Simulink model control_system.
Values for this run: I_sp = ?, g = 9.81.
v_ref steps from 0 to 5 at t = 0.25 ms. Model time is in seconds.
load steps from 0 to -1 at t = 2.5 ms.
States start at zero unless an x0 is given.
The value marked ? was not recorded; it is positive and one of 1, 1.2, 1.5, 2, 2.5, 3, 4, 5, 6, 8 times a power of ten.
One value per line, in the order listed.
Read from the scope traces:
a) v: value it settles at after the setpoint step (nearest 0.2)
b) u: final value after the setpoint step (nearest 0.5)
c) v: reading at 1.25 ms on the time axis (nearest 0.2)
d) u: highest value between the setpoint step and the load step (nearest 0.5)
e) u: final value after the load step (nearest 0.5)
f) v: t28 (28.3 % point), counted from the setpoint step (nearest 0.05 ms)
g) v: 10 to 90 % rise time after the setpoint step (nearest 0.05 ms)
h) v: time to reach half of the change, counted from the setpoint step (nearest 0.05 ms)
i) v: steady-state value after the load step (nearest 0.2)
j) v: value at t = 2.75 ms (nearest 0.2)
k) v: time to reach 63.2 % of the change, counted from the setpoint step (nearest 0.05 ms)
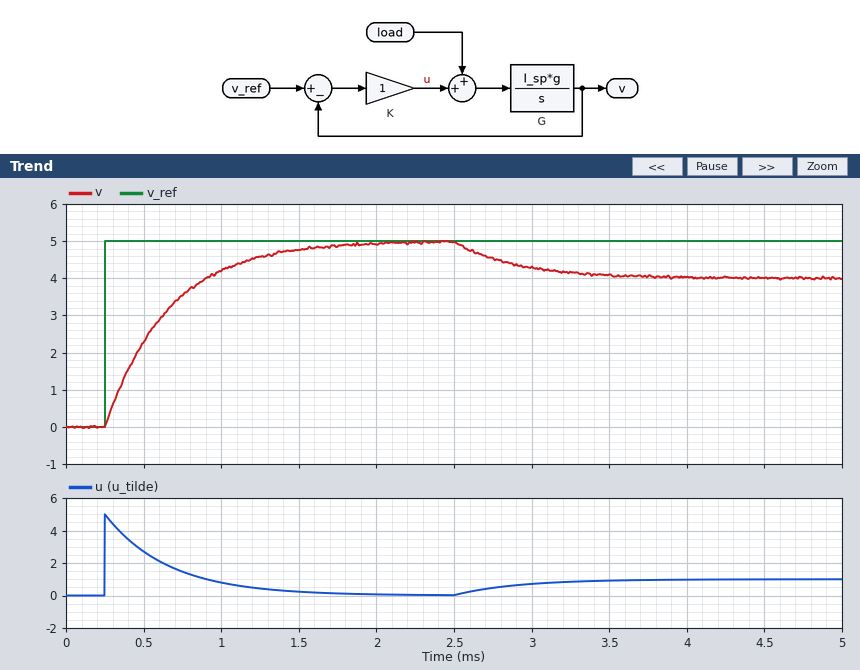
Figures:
5.0
0.0
4.6
5.0
1.0
0.15 ms
0.90 ms
0.30 ms
4.0
4.6
0.40 ms
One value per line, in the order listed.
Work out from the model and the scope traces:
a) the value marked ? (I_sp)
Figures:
250
